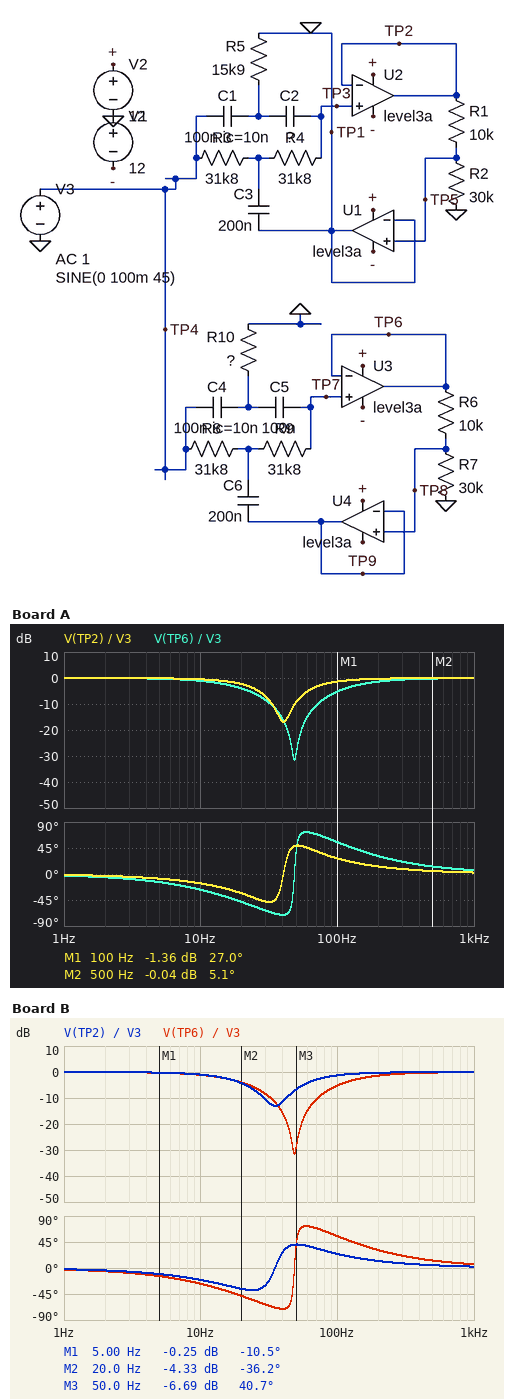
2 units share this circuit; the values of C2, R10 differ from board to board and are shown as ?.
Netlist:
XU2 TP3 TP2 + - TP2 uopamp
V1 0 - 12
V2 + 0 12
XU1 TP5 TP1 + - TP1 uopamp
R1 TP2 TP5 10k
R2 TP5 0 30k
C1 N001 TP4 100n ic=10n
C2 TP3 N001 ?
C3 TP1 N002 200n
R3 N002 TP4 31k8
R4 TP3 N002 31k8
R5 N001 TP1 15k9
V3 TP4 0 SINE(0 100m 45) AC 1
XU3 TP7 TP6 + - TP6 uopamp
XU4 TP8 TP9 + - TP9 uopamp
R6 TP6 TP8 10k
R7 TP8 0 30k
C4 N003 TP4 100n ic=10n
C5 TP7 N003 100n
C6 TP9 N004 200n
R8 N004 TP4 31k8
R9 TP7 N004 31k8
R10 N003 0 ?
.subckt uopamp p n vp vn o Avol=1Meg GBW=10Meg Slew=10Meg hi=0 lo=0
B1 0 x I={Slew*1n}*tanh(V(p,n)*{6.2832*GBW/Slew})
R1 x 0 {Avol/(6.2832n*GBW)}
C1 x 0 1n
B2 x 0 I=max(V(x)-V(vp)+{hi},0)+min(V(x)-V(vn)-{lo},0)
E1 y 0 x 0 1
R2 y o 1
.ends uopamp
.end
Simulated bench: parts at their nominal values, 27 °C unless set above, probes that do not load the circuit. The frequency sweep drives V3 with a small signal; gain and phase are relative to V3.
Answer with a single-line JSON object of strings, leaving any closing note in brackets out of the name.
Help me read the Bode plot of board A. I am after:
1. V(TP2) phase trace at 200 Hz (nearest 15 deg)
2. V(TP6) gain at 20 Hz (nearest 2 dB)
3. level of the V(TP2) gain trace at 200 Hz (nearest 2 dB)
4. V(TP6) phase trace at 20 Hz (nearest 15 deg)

{"V(TP2) phase trace at 200 Hz": "15 deg", "V(TP6) gain at 20 Hz": "-4 dB", "level of the V(TP2) gain trace at 200 Hz": "0 dB", "V(TP6) phase trace at 20 Hz": "-45 deg"}
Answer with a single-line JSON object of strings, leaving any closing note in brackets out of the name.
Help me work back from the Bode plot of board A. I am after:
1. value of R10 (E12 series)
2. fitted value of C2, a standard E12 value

{"value of R10": "18 kΩ", "fitted value of C2, a standard E12 value": "180 nF"}
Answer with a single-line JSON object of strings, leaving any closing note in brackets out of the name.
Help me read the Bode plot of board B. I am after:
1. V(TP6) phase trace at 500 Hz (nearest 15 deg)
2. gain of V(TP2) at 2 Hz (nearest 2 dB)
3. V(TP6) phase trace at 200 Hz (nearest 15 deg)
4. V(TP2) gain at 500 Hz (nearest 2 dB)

{"V(TP6) phase trace at 500 Hz": "15 deg", "gain of V(TP2) at 2 Hz": "0 dB", "V(TP6) phase trace at 200 Hz": "30 deg", "V(TP2) gain at 500 Hz": "0 dB"}
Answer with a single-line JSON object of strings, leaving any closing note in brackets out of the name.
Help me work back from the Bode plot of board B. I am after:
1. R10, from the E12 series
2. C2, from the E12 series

{"R10, from the E12 series": "18 kΩ", "C2, from the E12 series": "270 nF"}
